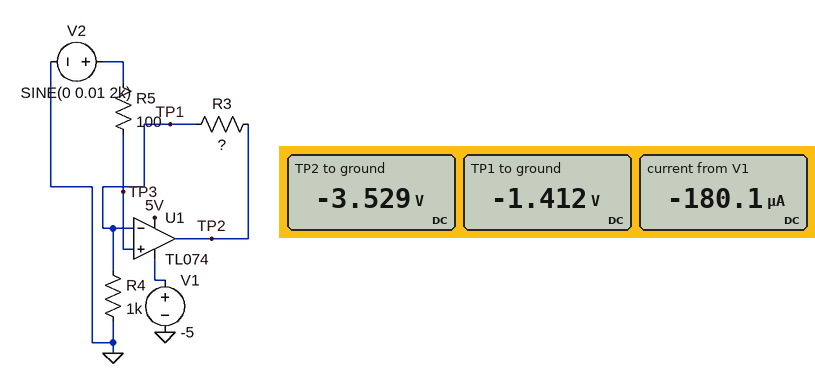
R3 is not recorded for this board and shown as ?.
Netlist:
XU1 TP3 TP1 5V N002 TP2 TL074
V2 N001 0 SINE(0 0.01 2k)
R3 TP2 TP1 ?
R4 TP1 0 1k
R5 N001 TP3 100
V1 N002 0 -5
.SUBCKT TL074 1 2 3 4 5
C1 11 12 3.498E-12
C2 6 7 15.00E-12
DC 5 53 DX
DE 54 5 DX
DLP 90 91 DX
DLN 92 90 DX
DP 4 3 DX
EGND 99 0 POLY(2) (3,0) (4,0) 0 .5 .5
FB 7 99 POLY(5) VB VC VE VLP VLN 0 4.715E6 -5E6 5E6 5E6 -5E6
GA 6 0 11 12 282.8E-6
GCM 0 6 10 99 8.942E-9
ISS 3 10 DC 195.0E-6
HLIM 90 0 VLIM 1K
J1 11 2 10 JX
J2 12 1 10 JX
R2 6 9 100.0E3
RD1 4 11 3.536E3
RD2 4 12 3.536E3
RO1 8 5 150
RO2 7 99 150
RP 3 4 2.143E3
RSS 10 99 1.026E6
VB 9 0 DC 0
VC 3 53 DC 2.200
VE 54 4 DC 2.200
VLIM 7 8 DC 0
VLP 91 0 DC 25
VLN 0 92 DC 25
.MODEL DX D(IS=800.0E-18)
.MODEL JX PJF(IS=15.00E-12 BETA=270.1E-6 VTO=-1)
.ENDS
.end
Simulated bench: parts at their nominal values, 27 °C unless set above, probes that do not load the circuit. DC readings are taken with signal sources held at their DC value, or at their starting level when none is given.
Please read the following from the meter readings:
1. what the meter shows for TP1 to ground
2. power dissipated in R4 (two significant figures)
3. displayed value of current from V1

-1.412 V
2.0 mW
-180.1 µA
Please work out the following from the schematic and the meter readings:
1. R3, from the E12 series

1.5 kΩ
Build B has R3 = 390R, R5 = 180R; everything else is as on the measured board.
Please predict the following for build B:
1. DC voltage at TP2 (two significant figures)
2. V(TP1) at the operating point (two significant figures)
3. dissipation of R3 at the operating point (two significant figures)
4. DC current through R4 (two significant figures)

-3.5 V
-2.5 V
2.5 mW
2.5 mA
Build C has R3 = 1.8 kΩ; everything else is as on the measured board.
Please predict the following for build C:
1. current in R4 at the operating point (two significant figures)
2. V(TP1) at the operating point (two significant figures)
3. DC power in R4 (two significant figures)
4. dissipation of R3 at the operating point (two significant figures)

1.3 mA
-1.3 V
1.6 mW
2.9 mW
